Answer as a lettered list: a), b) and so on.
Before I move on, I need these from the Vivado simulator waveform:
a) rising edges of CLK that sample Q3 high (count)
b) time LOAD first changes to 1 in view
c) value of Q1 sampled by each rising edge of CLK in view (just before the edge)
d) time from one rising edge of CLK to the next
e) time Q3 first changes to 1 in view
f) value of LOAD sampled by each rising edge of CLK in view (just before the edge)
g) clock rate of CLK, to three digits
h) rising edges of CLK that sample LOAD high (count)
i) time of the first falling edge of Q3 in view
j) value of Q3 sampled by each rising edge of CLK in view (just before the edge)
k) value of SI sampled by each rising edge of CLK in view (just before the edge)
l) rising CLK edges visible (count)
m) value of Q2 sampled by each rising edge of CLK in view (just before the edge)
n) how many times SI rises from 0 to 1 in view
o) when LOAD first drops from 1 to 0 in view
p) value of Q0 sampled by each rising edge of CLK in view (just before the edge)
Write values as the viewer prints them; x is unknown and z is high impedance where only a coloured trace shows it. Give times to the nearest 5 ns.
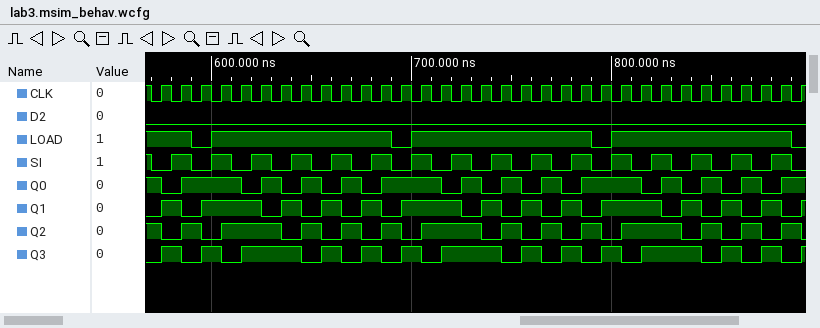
a) 19
b) 600 ns
c) 0 1 0 1 1 1 0 1 0 1 0 1 0 1 1 1 0 1 0 1 0 1 0 1 1 1 0 1 0 1 0 1 0
d) 10 ns
e) 575 ns
f) 1 1 0 1 1 1 1 1 1 1 1 1 0 1 1 1 1 1 1 1 1 1 0 1 1 1 1 1 1 1 1 1 0
g) 100 MHz
h) 29
i) 585 ns
j) 0 1 0 1 0 1 1 1 0 1 0 1 0 1 0 1 1 1 0 1 0 1 0 1 0 1 1 1 0 1 0 1 0
k) 0 1 0 1 0 1 0 1 0 1 0 1 0 1 0 1 0 1 0 1 0 1 0 1 0 1 0 1 0 1 0 1 0
l) 33
m) 1 0 1 0 1 1 1 0 1 0 1 0 1 0 1 1 1 0 1 0 1 0 1 0 1 1 1 0 1 0 1 0 1
n) 16
o) 590 ns
p) 1 0 1 1 1 0 1 0 1 0 1 0 1 1 1 0 1 0 1 0 1 0 1 1 1 0 1 0 1 0 1 0 1
